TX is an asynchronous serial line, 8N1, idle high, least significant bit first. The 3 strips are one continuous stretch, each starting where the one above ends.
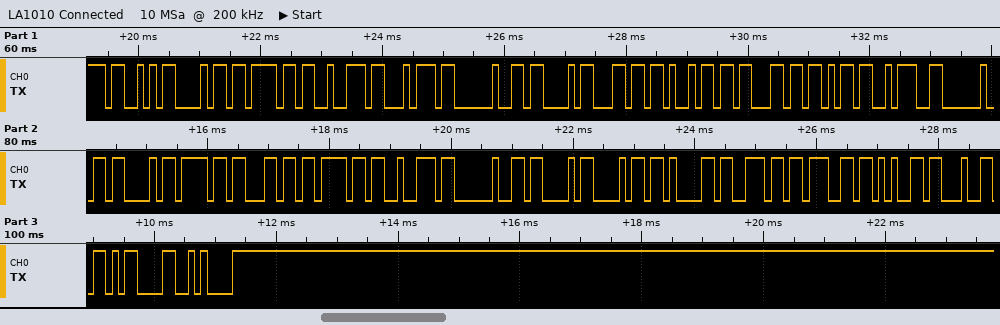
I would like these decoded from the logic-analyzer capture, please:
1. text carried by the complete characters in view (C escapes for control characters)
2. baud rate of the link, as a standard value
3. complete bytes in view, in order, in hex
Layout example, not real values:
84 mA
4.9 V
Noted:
"Short Click: Color Changed\r\n"
9600 baud
53 68 6F 72 74 20 43 6C 69 63 6B 3A 20 43 6F 6C 6F 72 20 43 68 61 6E 67 65 64 0D 0A
